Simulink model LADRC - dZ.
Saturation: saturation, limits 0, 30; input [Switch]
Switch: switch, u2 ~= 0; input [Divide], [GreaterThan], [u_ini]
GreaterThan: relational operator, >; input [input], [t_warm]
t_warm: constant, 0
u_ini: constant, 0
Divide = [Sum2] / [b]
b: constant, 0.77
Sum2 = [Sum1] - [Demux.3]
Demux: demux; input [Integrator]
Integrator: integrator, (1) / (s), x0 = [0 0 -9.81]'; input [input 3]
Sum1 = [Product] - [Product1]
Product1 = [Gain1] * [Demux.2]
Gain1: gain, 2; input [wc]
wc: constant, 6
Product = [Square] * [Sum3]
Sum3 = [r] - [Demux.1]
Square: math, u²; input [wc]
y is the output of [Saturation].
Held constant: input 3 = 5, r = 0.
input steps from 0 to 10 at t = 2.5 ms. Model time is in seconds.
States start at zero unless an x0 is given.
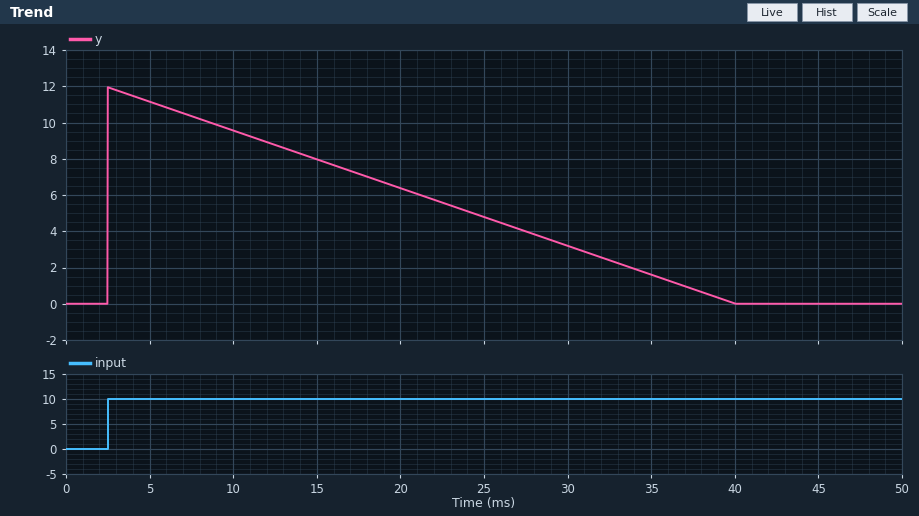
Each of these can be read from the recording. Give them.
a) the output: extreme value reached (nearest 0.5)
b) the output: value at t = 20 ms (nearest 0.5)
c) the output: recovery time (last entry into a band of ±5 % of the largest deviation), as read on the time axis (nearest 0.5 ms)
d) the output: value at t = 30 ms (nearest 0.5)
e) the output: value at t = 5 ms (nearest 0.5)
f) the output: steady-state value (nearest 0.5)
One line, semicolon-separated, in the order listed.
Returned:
12.0; 6.5; 38.0 ms; 3.0; 11.0; 0.0
